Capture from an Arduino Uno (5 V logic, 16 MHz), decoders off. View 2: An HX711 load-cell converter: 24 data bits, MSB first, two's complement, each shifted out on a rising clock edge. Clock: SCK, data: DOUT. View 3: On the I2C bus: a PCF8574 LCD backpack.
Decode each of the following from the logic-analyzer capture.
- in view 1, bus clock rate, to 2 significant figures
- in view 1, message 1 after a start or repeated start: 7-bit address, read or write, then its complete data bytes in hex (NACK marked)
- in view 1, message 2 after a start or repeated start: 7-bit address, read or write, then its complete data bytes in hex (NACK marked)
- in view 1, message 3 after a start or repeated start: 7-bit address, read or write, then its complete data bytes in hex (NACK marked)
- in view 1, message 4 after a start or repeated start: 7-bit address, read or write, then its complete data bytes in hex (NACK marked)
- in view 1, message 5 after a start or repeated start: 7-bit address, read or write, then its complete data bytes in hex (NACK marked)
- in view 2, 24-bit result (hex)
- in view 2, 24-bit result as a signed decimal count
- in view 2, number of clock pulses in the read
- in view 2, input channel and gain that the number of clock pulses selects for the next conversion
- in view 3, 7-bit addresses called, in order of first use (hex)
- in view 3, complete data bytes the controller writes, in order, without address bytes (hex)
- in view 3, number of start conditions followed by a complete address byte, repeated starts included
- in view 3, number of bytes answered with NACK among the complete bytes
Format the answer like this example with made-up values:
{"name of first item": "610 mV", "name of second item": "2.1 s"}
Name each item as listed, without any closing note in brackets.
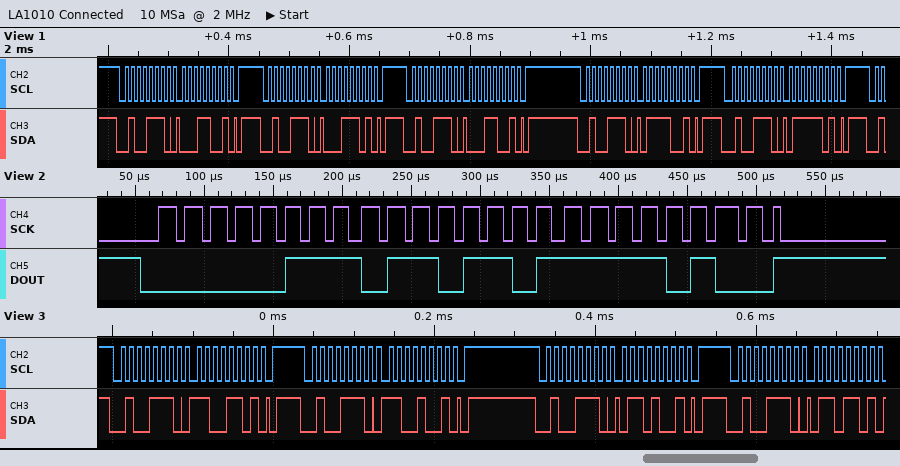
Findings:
{"in view 1, bus clock rate, to 2 significant figures": "100 kHz", "in view 1, message 1 after a start or repeated start: 7-bit address, read or write, then its complete data bytes in hex": "0x27 write: 19", "in view 1, message 2 after a start or repeated start: 7-bit address, read or write, then its complete data bytes in hex": "0x27 write: 1D", "in view 1, message 3 after a start or repeated start: 7-bit address, read or write, then its complete data bytes in hex": "0x27 write: 19", "in view 1, message 4 after a start or repeated start: 7-bit address, read or write, then its complete data bytes in hex": "0x27 write: 79", "in view 1, message 5 after a start or repeated start: 7-bit address, read or write, then its complete data bytes in hex": "0x27 write: 7D", "in view 2, 24-bit result": "0x076DF4", "in view 2, 24-bit result as a signed decimal count": "486900", "in view 2, number of clock pulses in the read": "25", "in view 2, input channel and gain that the number of clock pulses selects for the next conversion": "channel A, gain 128", "in view 3, 7-bit addresses called, in order of first use": "0x27", "in view 3, complete data bytes the controller writes, in order, without address bytes": "CD C9 69 6D", "in view 3, number of start conditions followed by a complete address byte, repeated starts included": "4", "in view 3, number of bytes answered with NACK among the complete bytes": "0"}
